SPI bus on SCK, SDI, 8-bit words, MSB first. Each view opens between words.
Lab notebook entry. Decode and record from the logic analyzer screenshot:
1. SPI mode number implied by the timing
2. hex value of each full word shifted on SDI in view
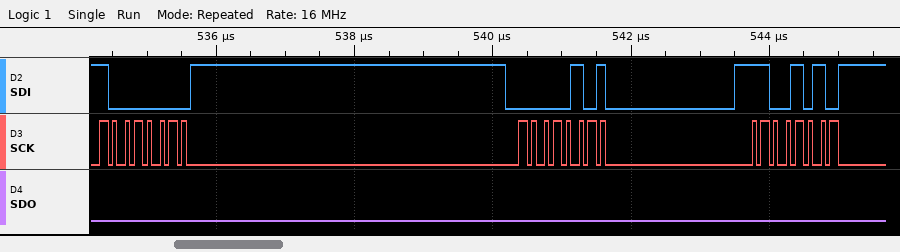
0
80, 05, CA
